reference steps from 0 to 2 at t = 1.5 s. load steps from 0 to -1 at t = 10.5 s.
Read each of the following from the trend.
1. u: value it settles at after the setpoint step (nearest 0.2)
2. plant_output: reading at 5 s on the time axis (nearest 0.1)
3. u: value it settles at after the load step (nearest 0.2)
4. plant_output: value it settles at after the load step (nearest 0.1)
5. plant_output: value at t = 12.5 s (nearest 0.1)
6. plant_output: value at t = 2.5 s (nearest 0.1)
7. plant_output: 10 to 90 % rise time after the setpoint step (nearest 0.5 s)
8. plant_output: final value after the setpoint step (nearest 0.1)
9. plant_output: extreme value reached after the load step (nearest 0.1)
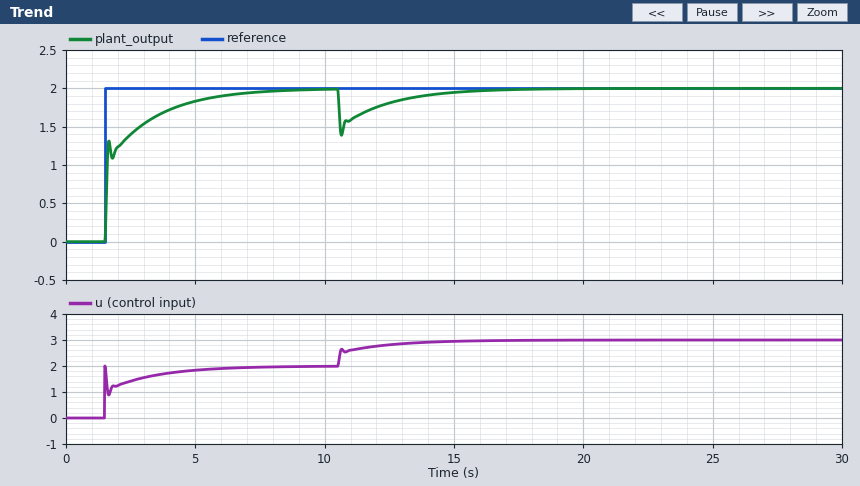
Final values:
2.0
1.8
3.0
2.0
1.8
1.4
3.0 s
2.0
1.4
